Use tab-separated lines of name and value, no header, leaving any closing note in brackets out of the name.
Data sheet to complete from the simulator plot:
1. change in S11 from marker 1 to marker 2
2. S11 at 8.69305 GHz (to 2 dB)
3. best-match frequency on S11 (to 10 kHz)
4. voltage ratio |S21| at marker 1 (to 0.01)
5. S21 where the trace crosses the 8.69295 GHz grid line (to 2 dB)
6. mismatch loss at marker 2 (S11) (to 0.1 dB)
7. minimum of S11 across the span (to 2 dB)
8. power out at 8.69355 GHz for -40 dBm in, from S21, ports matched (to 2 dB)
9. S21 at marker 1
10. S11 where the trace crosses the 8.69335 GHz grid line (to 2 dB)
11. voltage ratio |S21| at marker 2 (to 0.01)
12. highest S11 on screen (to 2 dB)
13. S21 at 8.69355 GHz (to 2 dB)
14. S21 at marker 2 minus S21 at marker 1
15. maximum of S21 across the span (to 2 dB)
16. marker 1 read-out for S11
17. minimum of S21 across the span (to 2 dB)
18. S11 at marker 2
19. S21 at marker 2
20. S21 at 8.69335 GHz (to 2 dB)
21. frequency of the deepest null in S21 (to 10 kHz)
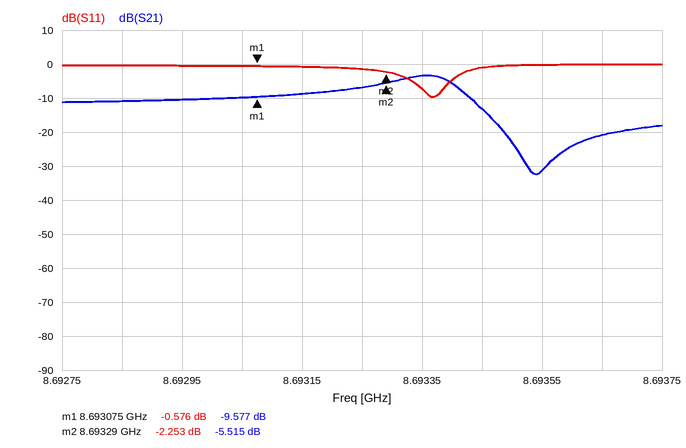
change in S11 from marker 1 to marker 2	-1.677 dB
S11 at 8.69305 GHz	0 dB
best-match frequency on S11	8.69337 GHz
voltage ratio |S21| at marker 1	0.33
S21 where the trace crosses the 8.69295 GHz grid line	-10 dB
mismatch loss at marker 2 (S11)	3.9 dB
minimum of S11 across the span	-10 dB
power out at 8.69355 GHz for -40 dBm in, from S21, ports matched	-72 dBm
S21 at marker 1	-9.577 dB
S11 where the trace crosses the 8.69335 GHz grid line	-8 dB
voltage ratio |S21| at marker 2	0.53
highest S11 on screen	0 dB
S21 at 8.69355 GHz	-32 dB
S21 at marker 2 minus S21 at marker 1	4.062 dB
maximum of S21 across the span	-4 dB
marker 1 read-out for S11	-0.576 dB
minimum of S21 across the span	-32 dB
S11 at marker 2	-2.253 dB
S21 at marker 2	-5.515 dB
S21 at 8.69335 GHz	-4 dB
frequency of the deepest null in S21	8.69354 GHz
